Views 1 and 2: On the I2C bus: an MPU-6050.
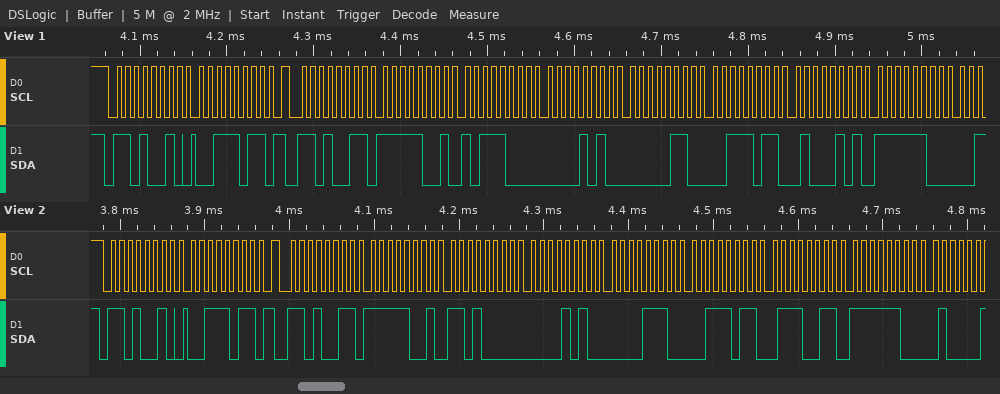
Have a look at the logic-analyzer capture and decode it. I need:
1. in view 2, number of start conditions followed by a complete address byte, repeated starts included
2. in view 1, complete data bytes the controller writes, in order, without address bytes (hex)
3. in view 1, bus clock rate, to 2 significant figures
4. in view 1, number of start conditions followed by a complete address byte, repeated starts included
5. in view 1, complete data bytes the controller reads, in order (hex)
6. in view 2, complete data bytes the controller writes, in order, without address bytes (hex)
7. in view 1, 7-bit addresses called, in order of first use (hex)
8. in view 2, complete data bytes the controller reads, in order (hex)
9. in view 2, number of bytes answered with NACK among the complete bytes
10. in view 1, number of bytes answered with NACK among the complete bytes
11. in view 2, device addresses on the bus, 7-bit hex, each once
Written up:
2
3B
100 kHz
2
F9 B8 0A 06 3B 45 FC
3B
0x69
F9 D0 0A 0E 3B 73 FC
0
0
0x69
